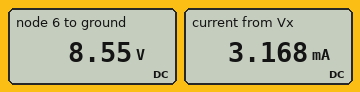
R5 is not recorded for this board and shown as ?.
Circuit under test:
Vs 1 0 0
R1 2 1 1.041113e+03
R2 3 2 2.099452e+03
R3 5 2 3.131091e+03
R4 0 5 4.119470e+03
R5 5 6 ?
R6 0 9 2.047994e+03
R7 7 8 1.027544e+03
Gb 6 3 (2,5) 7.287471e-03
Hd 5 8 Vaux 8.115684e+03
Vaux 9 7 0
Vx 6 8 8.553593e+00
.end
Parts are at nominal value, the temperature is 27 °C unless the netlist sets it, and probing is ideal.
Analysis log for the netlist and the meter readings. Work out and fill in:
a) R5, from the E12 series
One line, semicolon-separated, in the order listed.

2.7 kΩ
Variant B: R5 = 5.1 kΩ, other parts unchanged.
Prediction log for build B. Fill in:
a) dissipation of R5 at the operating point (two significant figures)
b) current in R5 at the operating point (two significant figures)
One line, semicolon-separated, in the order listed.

14 mW; 1.7 mA
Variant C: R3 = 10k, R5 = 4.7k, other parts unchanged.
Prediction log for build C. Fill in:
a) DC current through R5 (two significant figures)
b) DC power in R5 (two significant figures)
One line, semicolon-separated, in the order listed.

1.8 mA; 16 mW
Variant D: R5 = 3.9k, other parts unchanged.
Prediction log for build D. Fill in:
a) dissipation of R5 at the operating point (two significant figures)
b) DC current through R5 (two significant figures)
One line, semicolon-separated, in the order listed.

19 mW; 2.2 mA
